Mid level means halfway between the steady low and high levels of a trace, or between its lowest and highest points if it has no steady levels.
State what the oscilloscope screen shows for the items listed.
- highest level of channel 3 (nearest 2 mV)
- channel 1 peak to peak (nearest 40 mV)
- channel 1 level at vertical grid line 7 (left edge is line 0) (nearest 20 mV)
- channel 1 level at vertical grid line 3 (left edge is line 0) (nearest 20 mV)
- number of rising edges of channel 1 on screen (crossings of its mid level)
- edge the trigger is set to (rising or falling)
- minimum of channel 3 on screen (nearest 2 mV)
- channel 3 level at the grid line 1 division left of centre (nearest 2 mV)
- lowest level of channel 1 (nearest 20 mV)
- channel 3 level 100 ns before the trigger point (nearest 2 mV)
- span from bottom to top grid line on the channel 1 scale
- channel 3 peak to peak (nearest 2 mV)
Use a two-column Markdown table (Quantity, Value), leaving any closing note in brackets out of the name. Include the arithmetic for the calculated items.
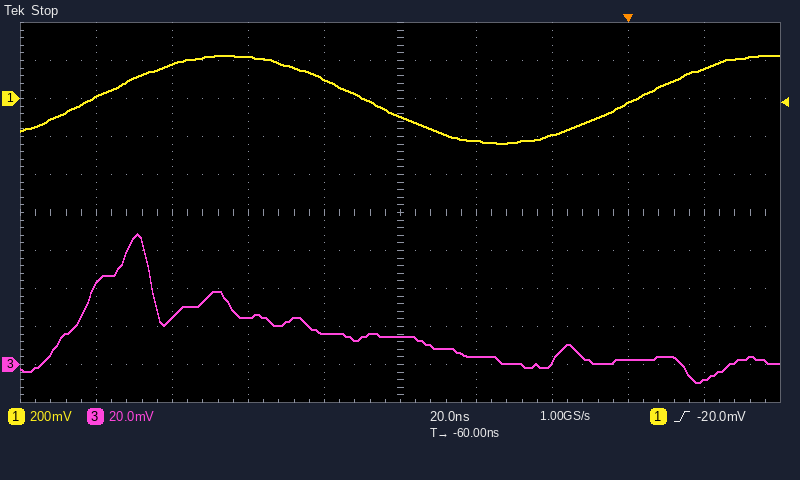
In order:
| Quantity | Value |
|---|---|
| highest level of channel 3 | 68 mV |
| channel 1 peak to peak | 480 mV |
| channel 1 level at vertical grid line 7 (left edge is line 0) | -200 mV |
| channel 1 level at vertical grid line 3 (left edge is line 0) | 220 mV |
| number of rising edges of channel 1 on screen | 2 |
| edge the trigger is set to | rising |
| minimum of channel 3 on screen | -10 mV |
| channel 3 level at the grid line 1 division left of centre | 16 mV |
| lowest level of channel 1 | -240 mV |
| channel 3 level 100 ns before the trigger point | 24 mV |
| span from bottom to top grid line on the channel 1 scale | 2 V |
| channel 3 peak to peak | 68 mV − (-10 mV) = 78 mV |
